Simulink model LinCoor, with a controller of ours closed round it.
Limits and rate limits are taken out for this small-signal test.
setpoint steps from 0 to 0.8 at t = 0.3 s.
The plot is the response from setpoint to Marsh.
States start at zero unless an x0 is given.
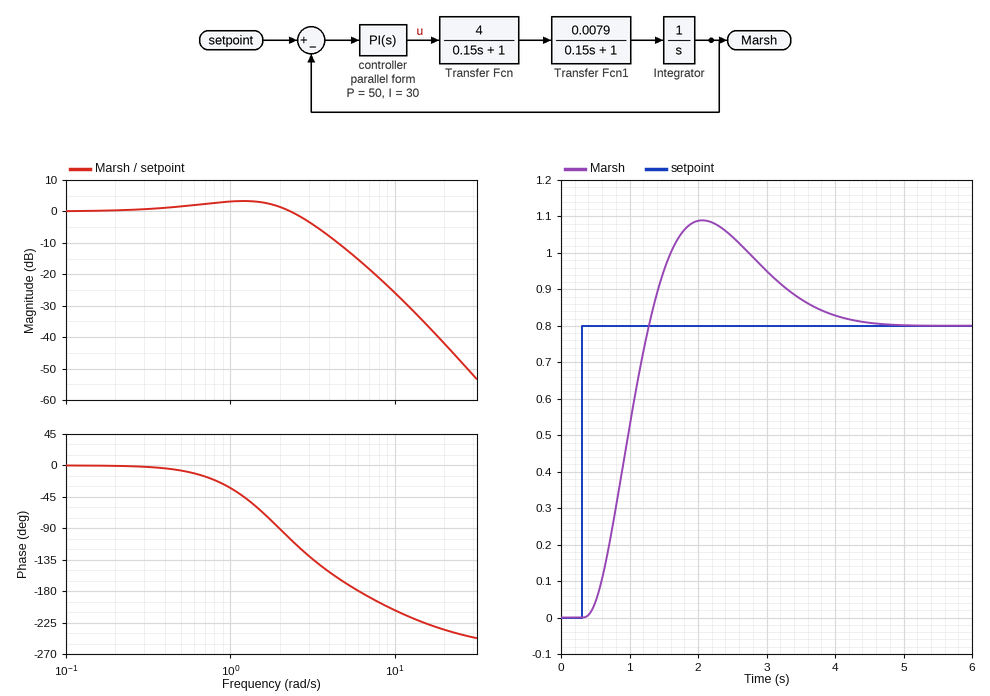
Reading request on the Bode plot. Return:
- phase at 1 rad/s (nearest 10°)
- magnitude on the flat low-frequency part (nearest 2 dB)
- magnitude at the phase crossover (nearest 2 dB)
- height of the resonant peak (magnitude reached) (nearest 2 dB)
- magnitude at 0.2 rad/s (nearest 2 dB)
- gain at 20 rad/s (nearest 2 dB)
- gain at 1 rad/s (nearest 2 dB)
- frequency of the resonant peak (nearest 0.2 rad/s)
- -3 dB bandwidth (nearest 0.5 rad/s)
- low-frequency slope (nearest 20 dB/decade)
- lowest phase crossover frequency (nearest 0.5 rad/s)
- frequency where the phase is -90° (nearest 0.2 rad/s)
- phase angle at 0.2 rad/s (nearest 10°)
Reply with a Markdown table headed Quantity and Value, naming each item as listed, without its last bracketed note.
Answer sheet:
| Quantity | Value |
|---|---|
| phase at 1 rad/s | -30° |
| magnitude on the flat low-frequency part | 0 dB |
| magnitude at the phase crossover | -16 dB |
| height of the resonant peak (magnitude reached) | 4 dB |
| magnitude at 0.2 rad/s | 0 dB |
| gain at 20 rad/s | -42 dB |
| gain at 1 rad/s | 4 dB |
| frequency of the resonant peak | 1.2 rad/s |
| -3 dB bandwidth | 3.0 rad/s |
| low-frequency slope | 0 dB/decade |
| lowest phase crossover frequency | 6.0 rad/s |
| frequency where the phase is -90° | 2.0 rad/s |
| phase angle at 0.2 rad/s | 0° |
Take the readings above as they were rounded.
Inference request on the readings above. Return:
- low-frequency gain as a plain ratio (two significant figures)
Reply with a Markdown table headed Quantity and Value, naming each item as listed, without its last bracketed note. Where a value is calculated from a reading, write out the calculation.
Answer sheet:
| Quantity | Value |
|---|---|
| low-frequency gain as a plain ratio | 10^(0 / 20) = 1.0 |
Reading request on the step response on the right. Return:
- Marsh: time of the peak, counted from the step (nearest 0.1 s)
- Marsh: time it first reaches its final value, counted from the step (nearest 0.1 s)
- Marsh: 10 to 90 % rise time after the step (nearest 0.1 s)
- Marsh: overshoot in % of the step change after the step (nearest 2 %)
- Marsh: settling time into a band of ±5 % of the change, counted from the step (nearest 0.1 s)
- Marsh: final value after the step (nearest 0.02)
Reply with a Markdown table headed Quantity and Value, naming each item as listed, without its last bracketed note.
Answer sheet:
| Quantity | Value |
|---|---|
| Marsh: time of the peak, counted from the step | 1.8 s |
| Marsh: time it first reaches its final value, counted from the step | 1.0 s |
| Marsh: 10 to 90 % rise time after the step | 0.6 s |
| Marsh: overshoot in % of the step change after the step | 36 % |
| Marsh: settling time into a band of ±5 % of the change, counted from the step | 3.5 s |
| Marsh: final value after the step | 0.80 |
